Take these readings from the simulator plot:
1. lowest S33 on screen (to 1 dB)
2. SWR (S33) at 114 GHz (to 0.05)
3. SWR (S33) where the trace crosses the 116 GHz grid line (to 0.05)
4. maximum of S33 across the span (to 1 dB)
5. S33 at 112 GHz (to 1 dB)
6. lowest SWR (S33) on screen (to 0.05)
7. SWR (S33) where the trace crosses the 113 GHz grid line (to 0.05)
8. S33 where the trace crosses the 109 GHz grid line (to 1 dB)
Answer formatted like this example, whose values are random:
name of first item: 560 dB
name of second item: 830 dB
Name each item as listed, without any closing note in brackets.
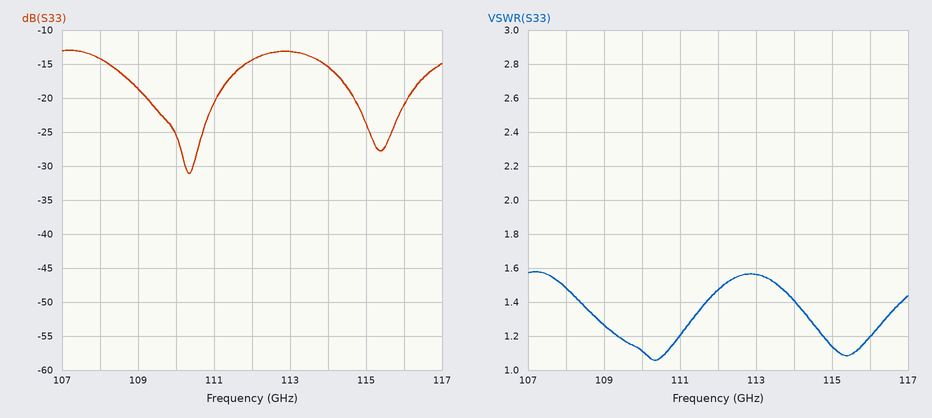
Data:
lowest S33 on screen: -31 dB
SWR (S33) at 114 GHz: 1.40
SWR (S33) where the trace crosses the 116 GHz grid line: 1.20
maximum of S33 across the span: -13 dB
S33 at 112 GHz: -14 dB
lowest SWR (S33) on screen: 1.05
SWR (S33) where the trace crosses the 113 GHz grid line: 1.55
S33 where the trace crosses the 109 GHz grid line: -19 dB
